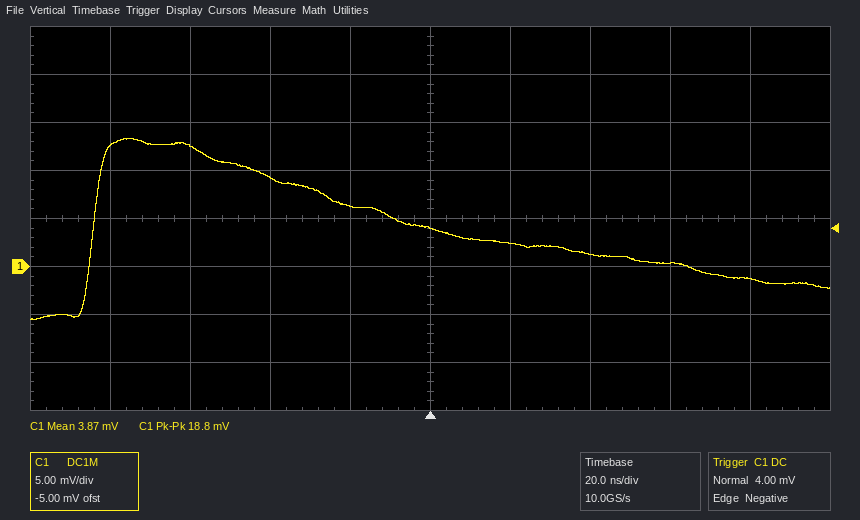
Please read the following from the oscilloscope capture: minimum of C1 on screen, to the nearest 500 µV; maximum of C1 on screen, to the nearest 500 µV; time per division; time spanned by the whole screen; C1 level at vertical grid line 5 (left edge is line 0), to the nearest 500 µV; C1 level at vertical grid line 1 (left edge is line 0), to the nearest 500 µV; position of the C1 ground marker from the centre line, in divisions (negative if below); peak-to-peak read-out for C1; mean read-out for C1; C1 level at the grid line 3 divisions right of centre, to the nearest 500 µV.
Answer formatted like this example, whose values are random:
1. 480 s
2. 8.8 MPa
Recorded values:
1. -5.5 mV
2. 13.5 mV
3. 20 ns
4. 200 ns
5. 4.0 mV
6. 12.5 mV
7. -1.0 div
8. 18.8 mV
9. 3.87 mV
10. 500 µV
